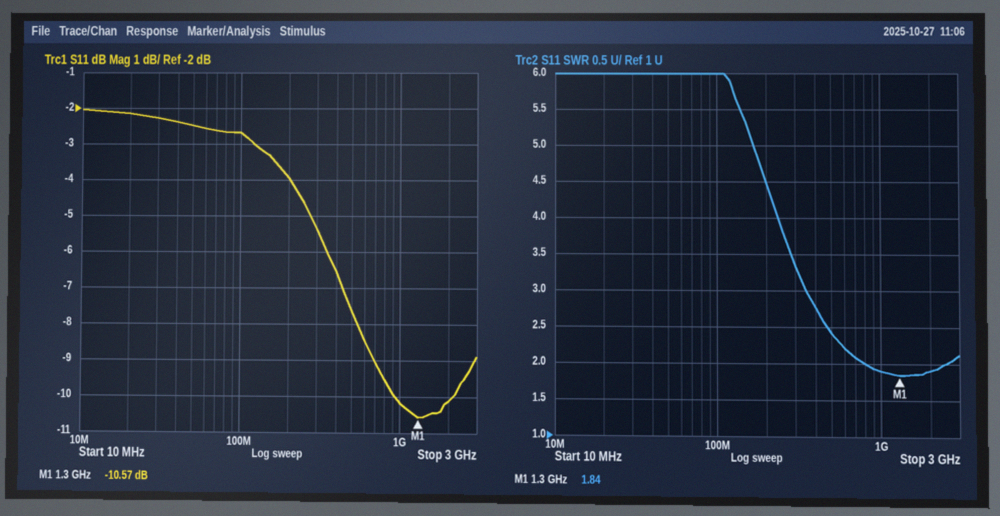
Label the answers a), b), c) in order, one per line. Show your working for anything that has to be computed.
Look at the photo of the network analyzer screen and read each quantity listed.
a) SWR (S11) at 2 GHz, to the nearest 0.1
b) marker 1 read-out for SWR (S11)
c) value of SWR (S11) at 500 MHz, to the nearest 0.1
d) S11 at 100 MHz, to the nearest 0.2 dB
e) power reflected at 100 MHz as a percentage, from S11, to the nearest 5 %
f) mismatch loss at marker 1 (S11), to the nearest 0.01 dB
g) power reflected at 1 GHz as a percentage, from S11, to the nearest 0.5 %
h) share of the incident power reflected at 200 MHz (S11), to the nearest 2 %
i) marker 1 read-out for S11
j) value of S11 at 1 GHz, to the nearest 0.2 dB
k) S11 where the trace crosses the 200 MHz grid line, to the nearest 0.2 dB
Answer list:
a) 1.9
b) 1.84
c) 2.4
d) -2.6 dB
e) 10^(-2.6/10) ≈ 55 %
f) −10 log10(1 − 10^(-10.57/10)) ≈ 0.40 dB
g) 10^(-10.2/10) ≈ 9.5 %
h) 10^(-4/10) ≈ 40 %
i) -10.57 dB
j) -10.2 dB
k) -4.0 dB
